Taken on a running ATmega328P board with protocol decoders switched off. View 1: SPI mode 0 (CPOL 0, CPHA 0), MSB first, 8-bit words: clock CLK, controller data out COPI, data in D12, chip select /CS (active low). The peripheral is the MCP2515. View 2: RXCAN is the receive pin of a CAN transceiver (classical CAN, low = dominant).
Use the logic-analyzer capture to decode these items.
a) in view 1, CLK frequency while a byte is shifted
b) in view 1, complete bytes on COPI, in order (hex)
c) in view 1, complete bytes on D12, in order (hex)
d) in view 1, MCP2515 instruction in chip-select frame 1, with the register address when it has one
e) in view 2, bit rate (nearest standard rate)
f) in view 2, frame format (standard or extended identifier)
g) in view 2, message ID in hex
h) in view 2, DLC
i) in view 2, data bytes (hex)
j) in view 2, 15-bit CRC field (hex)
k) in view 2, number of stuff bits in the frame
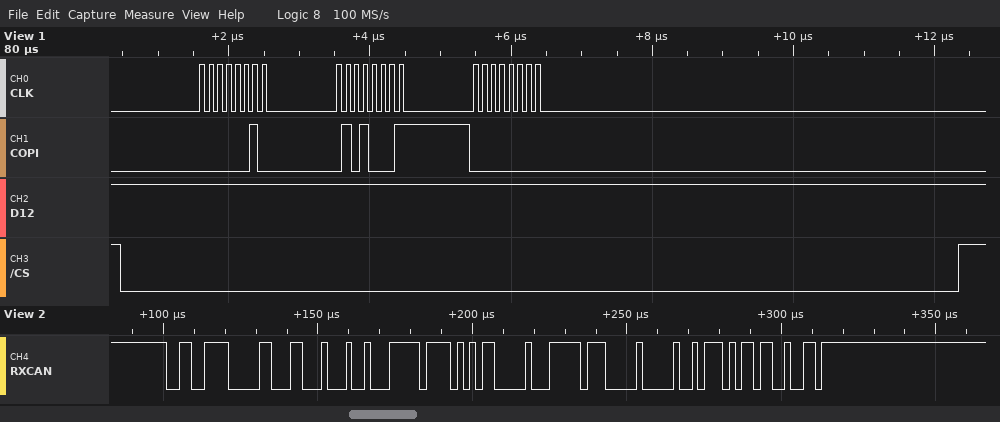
8 MHz
0x02 0x51 0x00
0xFF 0xFF 0xFF
WRITE 0x51
500 kbit/s
standard
0x33C
8
C4 48 FF AB 00 FF 00 0B
0x56C9
6
